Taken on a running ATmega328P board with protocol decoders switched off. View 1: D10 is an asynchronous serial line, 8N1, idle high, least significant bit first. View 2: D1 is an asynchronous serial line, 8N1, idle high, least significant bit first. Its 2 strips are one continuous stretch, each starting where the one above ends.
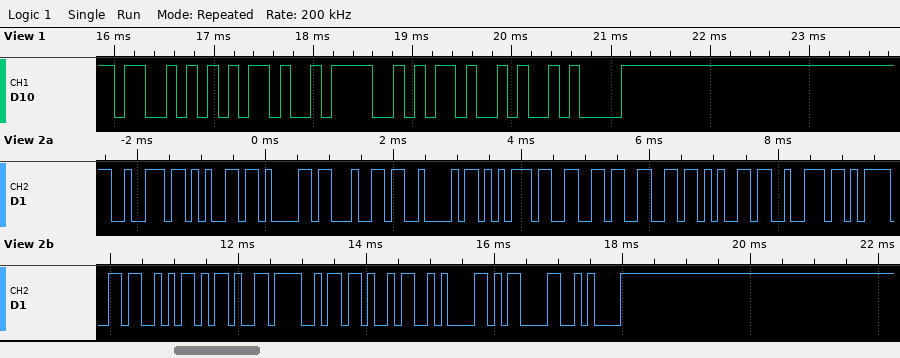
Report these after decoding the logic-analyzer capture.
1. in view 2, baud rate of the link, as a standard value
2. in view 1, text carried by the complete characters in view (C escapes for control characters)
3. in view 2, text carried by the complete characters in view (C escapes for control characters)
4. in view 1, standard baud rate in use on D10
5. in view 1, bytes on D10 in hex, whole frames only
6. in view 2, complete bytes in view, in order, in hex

9600 baud
"S-OK\n"
"readBuffer=S-OK\n\r\n"
9600 baud
0x53 0x2D 0x4F 0x4B 0x0A
72 65 61 64 42 75 66 66 65 72 3D 53 2D 4F 4B 0A 0D 0A
